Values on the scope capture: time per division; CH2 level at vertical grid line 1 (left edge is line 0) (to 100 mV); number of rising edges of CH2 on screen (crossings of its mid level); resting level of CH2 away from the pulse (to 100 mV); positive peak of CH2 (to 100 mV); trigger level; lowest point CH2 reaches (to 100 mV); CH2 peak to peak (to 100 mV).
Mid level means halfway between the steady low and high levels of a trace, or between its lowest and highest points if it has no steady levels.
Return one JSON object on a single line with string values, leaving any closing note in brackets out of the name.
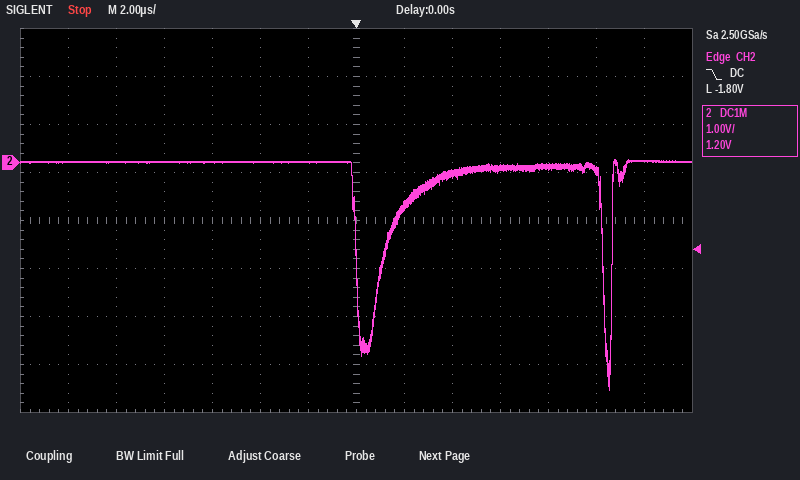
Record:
{"time per division": "2 µs", "CH2 level at vertical grid line 1 (left edge is line 0)": "0.0 V", "number of rising edges of CH2 on screen": "2", "resting level of CH2 away from the pulse": "0.0 V", "positive peak of CH2": "100 mV", "trigger level": "-1.80 V", "lowest point CH2 reaches": "-4.7 V", "CH2 peak to peak": "4.8 V"}
